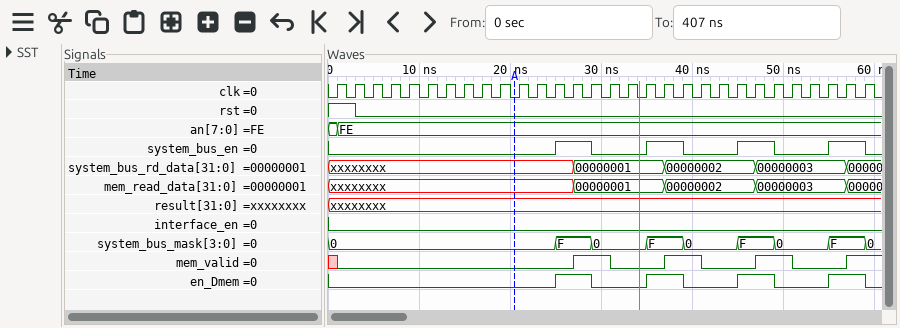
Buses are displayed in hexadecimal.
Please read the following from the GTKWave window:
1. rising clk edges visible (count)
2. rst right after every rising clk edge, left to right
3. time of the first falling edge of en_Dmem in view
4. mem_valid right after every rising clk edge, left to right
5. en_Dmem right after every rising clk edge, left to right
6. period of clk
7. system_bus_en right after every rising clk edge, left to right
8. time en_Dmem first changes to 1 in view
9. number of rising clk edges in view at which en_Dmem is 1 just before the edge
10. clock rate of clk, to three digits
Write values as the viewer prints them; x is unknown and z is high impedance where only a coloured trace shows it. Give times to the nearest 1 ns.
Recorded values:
30
1 0 0 0 0 0 0 0 0 0 0 0 0 0 0 0 0 0 0 0 0 0 0 0 0 0 0 0 0 0
29 ns
0 0 0 0 0 0 0 0 0 0 0 0 0 1 1 0 0 0 1 1 0 0 0 1 1 0 0 0 1 1
0 0 0 0 0 0 0 0 0 0 0 0 1 1 0 0 0 1 1 0 0 0 1 1 0 0 0 1 1 0
2 ns
0 0 0 0 0 0 0 0 0 0 0 0 1 1 0 0 0 1 1 0 0 0 1 1 0 0 0 1 1 0
25 ns
8
500 MHz
